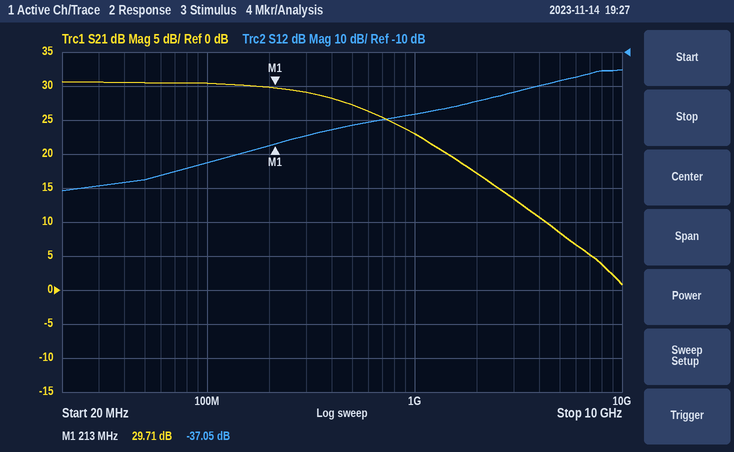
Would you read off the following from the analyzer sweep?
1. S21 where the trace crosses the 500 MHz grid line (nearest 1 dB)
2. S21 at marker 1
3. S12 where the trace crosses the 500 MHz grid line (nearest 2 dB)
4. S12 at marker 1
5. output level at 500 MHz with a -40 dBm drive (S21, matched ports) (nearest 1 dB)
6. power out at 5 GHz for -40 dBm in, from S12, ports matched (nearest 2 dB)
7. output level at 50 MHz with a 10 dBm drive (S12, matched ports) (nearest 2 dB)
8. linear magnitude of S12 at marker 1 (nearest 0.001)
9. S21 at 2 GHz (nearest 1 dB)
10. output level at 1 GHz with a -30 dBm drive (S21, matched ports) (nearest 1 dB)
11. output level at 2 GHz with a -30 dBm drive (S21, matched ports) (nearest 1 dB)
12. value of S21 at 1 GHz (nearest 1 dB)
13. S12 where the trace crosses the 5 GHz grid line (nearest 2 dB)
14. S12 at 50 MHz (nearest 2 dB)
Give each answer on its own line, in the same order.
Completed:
27 dB
29.71 dB
-32 dB
-37.05 dB
-13 dBm
-58 dBm
-38 dBm
0.014
17 dB
-7 dBm
-13 dBm
23 dB
-18 dB
-48 dB
